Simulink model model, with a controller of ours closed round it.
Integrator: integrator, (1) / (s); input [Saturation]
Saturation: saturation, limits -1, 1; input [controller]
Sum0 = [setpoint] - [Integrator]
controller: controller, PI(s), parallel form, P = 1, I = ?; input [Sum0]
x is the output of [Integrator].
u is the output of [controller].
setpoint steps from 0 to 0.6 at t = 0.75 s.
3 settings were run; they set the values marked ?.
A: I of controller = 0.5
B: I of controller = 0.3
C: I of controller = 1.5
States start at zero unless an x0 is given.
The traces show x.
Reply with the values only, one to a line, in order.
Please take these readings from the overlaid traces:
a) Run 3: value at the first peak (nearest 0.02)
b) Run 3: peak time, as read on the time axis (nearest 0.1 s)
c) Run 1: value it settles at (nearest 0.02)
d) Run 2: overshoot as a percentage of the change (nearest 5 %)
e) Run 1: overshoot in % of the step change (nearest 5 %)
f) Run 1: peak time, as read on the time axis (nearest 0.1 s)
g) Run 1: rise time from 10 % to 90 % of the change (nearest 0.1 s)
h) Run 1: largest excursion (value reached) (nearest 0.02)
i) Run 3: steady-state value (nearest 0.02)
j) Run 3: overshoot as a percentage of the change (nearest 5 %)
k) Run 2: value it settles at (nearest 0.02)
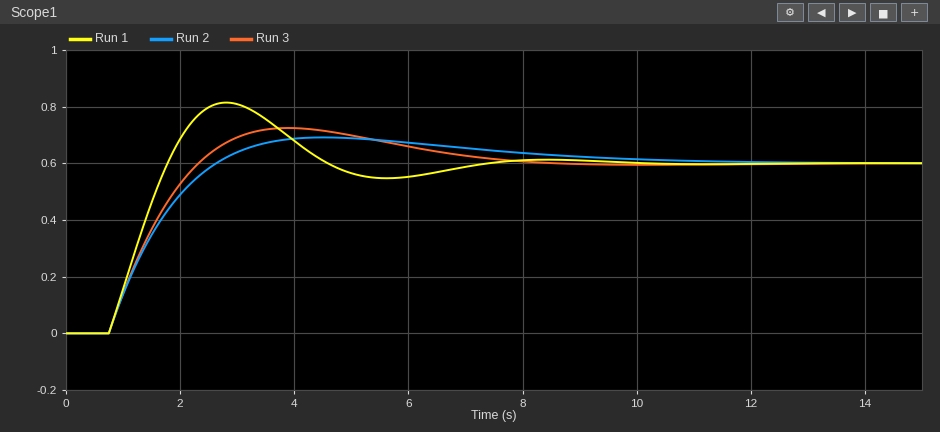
0.72
3.9 s
0.60
15 %
35 %
2.8 s
0.8 s
0.82
0.60
20 %
0.60
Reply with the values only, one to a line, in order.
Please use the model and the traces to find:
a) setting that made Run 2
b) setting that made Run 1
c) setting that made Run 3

B
C
A
